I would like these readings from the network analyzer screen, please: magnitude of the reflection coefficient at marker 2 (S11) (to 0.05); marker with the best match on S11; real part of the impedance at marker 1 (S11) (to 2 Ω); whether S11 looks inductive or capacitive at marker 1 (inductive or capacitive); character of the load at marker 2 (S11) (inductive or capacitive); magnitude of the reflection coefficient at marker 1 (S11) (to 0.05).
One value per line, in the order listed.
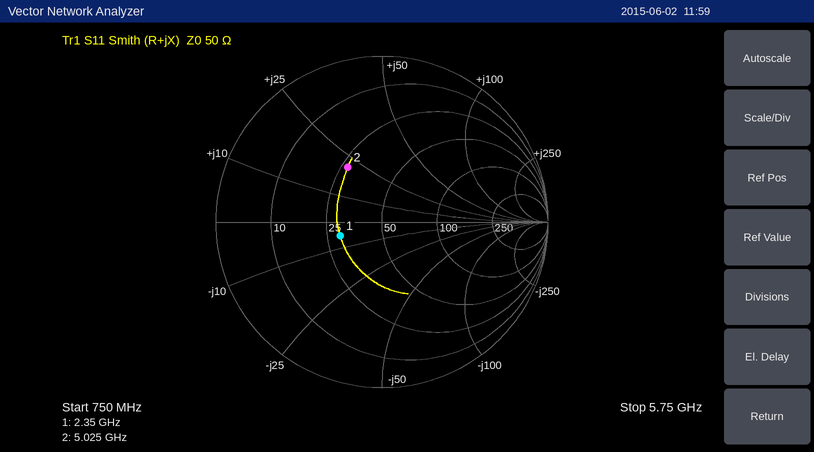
0.40
marker 1
30 Ω
capacitive
inductive
0.25
